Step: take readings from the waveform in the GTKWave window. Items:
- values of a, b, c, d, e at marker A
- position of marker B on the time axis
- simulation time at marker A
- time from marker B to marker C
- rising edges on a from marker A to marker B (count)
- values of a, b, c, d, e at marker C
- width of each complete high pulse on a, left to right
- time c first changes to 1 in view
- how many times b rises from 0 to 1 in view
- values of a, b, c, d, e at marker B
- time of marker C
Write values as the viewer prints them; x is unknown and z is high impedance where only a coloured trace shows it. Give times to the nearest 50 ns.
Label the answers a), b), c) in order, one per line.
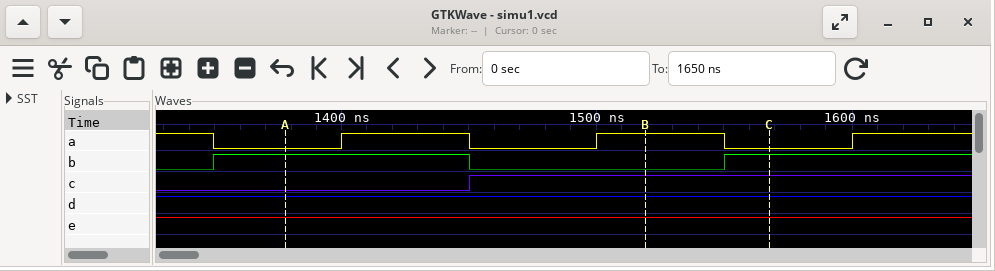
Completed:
a) a=0, b=1, c=0, d=1, e=1
b) 1500 ns
c) 1400 ns
d) 50 ns
e) 2
f) a=0, b=1, c=1, d=1, e=1
g) 50 ns, 50 ns
h) 1450 ns
i) 2
j) a=1, b=0, c=1, d=1, e=1
k) 1550 ns
